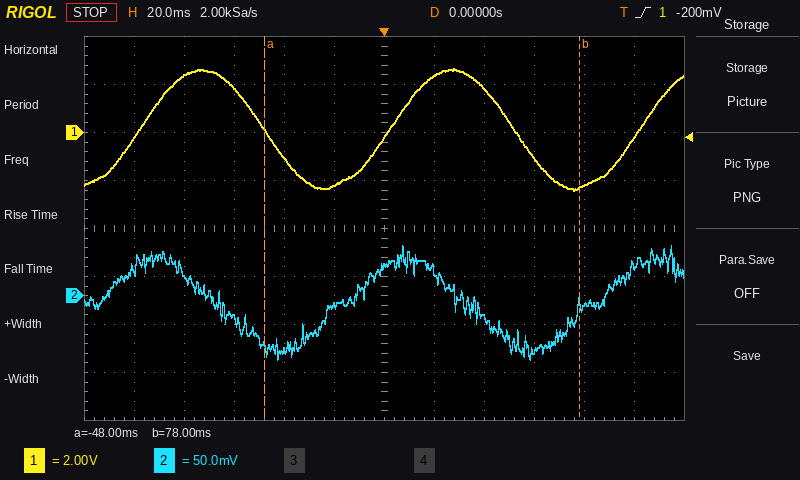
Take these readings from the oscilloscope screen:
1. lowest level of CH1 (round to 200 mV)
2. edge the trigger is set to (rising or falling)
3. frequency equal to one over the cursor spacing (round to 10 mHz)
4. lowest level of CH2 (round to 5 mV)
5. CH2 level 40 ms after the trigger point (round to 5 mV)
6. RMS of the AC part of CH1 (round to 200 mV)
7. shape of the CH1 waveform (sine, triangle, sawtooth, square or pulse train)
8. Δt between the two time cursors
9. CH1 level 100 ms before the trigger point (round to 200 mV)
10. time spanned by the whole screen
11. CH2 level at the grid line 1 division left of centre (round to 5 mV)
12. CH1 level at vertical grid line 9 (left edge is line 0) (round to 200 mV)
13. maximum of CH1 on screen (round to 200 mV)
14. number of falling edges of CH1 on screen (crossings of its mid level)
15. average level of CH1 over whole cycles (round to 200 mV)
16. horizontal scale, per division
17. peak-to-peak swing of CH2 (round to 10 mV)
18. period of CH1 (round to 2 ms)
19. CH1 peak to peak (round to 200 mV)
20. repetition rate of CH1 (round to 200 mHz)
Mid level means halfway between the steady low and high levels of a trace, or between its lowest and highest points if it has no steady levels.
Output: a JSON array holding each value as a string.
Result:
["-2.4 V", "rising", "7.94 Hz", "-65 mV", "-25 mV", "1.8 V", "sine", "126 ms", "-200 mV", "240 ms", "-10 mV", "-1.0 V", "2.6 V", "2", "200 mV", "20 ms", "120 mV", "100 ms", "5.0 V", "10.0 Hz"]
